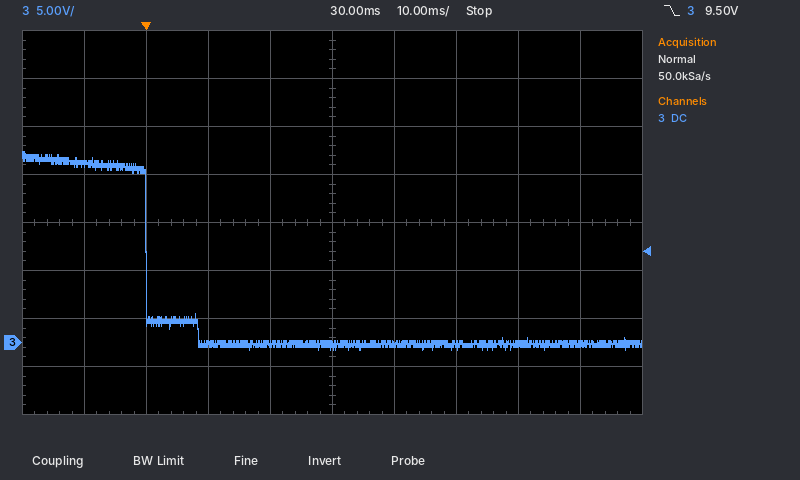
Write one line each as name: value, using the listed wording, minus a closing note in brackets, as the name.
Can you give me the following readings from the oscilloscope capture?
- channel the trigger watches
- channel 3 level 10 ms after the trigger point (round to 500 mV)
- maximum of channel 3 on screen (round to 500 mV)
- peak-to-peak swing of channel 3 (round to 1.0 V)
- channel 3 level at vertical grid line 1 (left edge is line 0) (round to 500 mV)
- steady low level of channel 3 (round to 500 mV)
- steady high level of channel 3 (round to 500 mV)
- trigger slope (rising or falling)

channel the trigger watches: channel 3
channel 3 level 10 ms after the trigger point: 0.0 V
maximum of channel 3 on screen: 20.0 V
peak-to-peak swing of channel 3: 21.0 V
channel 3 level at vertical grid line 1 (left edge is line 0): 18.5 V
steady low level of channel 3: 0.0 V
steady high level of channel 3: 18.5 V
trigger slope: falling
